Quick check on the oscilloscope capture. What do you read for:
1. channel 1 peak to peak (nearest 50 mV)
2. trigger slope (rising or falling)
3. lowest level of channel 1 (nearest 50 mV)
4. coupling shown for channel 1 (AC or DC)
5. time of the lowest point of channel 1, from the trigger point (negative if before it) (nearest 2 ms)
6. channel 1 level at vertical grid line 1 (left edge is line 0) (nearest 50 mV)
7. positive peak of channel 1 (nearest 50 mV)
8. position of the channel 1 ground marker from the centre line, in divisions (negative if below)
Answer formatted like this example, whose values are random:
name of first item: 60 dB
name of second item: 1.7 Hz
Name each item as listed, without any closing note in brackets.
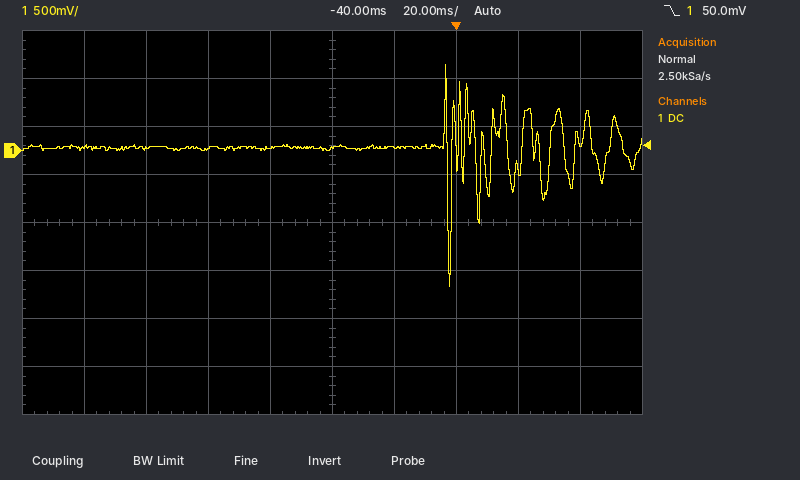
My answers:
channel 1 peak to peak: 2.30 V
trigger slope: falling
lowest level of channel 1: -1.40 V
coupling shown for channel 1: DC
time of the lowest point of channel 1, from the trigger point (negative if before it): -2 ms
channel 1 level at vertical grid line 1 (left edge is line 0): 50 mV
positive peak of channel 1: 900 mV
position of the channel 1 ground marker from the centre line, in divisions: +1.5 div
